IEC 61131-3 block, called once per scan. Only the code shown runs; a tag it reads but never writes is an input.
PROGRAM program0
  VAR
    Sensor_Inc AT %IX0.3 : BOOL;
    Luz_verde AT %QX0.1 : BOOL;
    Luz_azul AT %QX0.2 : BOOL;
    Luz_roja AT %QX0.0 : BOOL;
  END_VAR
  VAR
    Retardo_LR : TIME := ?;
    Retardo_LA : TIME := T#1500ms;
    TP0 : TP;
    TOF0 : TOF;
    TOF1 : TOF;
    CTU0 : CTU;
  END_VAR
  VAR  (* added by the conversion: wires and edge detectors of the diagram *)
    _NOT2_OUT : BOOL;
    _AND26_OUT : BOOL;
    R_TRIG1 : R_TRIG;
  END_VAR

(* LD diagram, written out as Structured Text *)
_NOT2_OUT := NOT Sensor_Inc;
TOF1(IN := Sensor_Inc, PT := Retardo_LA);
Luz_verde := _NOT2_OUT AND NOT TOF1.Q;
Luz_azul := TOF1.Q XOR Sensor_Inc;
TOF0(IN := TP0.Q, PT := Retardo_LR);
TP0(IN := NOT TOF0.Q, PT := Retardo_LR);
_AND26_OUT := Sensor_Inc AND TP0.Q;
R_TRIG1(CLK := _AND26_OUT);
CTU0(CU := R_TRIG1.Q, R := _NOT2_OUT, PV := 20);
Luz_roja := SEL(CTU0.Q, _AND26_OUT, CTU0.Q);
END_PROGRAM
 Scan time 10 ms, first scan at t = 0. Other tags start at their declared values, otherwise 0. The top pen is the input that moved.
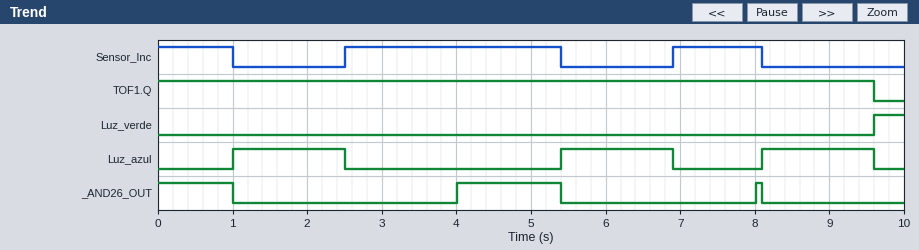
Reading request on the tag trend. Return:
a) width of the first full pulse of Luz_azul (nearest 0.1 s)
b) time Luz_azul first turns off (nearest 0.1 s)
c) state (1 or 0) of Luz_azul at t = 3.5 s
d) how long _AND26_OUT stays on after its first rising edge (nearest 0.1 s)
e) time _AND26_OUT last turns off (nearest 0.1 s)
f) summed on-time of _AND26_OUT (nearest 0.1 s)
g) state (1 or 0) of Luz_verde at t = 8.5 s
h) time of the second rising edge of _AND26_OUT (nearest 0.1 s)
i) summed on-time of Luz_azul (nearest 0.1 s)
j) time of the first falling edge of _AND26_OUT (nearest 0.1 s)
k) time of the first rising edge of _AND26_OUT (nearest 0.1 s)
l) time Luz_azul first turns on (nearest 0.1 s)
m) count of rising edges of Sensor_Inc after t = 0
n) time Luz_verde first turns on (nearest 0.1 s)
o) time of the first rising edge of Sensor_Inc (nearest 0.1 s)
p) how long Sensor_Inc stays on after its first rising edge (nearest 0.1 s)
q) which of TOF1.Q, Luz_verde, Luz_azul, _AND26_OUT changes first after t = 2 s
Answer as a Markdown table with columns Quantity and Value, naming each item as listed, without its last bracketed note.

| Quantity | Value |
|---|---|
| width of the first full pulse of Luz_azul | 1.5 s |
| time Luz_azul first turns off | 2.5 s |
| state (1 or 0) of Luz_azul at t = 3.5 s | 0 |
| how long _AND26_OUT stays on after its first rising edge | 1.4 s |
| time _AND26_OUT last turns off | 8.1 s |
| summed on-time of _AND26_OUT | 2.5 s |
| state (1 or 0) of Luz_verde at t = 8.5 s | 0 |
| time of the second rising edge of _AND26_OUT | 8.0 s |
| summed on-time of Luz_azul | 4.5 s |
| time of the first falling edge of _AND26_OUT | 1.0 s |
| time of the first rising edge of _AND26_OUT | 4.0 s |
| time Luz_azul first turns on | 1.0 s |
| count of rising edges of Sensor_Inc after t = 0 | 2 |
| time Luz_verde first turns on | 9.6 s |
| time of the first rising edge of Sensor_Inc | 2.5 s |
| how long Sensor_Inc stays on after its first rising edge | 2.9 s |
| which of TOF1.Q, Luz_verde, Luz_azul, _AND26_OUT changes first after t = 2 s | Luz_azul |
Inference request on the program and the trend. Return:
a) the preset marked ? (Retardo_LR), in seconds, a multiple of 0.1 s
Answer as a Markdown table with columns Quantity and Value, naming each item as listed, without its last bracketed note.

| Quantity | Value |
|---|---|
| the preset marked ? (Retardo_LR), in seconds, a multiple of 0.1 s | 2.0 s |
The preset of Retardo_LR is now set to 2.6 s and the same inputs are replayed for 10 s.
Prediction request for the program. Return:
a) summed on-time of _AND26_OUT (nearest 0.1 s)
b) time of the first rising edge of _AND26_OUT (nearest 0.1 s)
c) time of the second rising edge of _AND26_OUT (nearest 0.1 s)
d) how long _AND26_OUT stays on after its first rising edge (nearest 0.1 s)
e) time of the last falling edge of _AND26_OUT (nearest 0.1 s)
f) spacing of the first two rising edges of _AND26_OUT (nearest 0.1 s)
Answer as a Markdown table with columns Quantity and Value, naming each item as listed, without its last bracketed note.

| Quantity | Value |
|---|---|
| summed on-time of _AND26_OUT | 2.2 s |
| time of the first rising edge of _AND26_OUT | 2.5 s |
| time of the second rising edge of _AND26_OUT | 5.2 s |
| how long _AND26_OUT stays on after its first rising edge | 0.1 s |
| time of the last falling edge of _AND26_OUT | 7.8 s |
| spacing of the first two rising edges of _AND26_OUT | 2.7 s |
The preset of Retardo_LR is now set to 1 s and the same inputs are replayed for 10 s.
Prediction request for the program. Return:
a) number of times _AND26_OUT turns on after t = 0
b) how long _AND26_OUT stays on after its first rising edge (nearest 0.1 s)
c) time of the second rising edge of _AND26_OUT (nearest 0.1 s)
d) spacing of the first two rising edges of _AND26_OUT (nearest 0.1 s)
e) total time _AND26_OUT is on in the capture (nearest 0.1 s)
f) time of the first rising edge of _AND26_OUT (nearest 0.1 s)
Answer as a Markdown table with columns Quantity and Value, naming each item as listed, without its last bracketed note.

| Quantity | Value |
|---|---|
| number of times _AND26_OUT turns on after t = 0 | 4 |
| how long _AND26_OUT stays on after its first rising edge | 0.5 s |
| time of the second rising edge of _AND26_OUT | 4.0 s |
| spacing of the first two rising edges of _AND26_OUT | 1.5 s |
| total time _AND26_OUT is on in the capture | 2.7 s |
| time of the first rising edge of _AND26_OUT | 2.5 s |
